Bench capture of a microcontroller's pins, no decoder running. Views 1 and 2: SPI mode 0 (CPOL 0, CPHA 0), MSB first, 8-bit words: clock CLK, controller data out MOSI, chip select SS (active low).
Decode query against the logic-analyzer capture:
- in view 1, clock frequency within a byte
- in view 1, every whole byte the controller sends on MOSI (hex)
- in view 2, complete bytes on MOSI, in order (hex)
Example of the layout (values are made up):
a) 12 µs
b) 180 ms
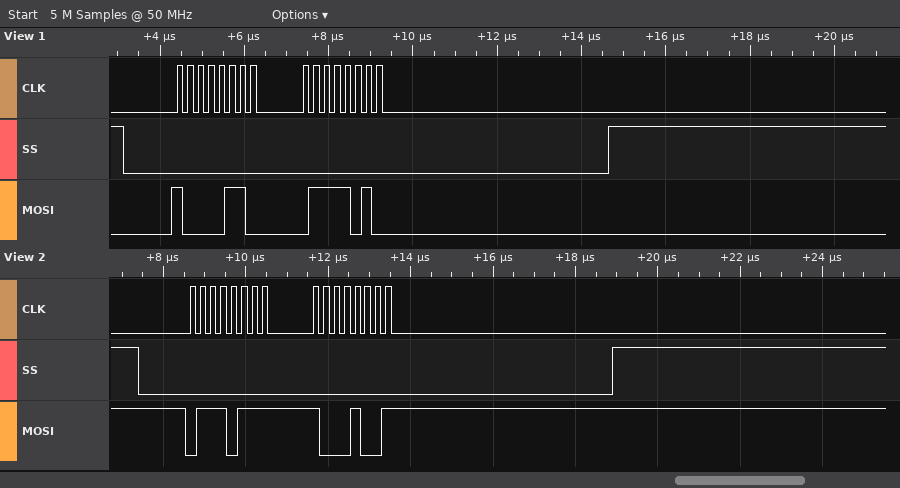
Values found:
a) 4 MHz
b) 0x86 0x7A
c) 0x77 0x89
